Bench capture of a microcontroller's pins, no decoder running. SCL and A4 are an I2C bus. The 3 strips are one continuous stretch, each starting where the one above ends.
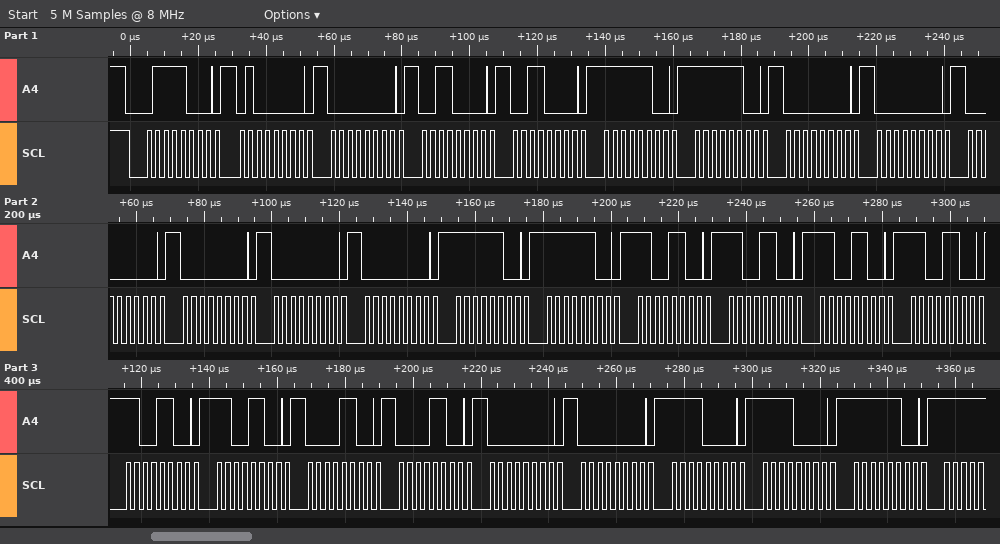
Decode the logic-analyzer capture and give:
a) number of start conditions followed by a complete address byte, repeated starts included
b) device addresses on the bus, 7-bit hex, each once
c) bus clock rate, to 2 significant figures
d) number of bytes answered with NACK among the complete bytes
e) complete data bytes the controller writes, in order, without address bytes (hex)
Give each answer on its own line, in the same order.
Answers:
1
0x3C
400 kHz
0
40 00 30 30 FC FC 00 00 00 00 00 00 FC FC CC CC CC CC CC CC 0C 0C 00 00 F0 F0 FC
